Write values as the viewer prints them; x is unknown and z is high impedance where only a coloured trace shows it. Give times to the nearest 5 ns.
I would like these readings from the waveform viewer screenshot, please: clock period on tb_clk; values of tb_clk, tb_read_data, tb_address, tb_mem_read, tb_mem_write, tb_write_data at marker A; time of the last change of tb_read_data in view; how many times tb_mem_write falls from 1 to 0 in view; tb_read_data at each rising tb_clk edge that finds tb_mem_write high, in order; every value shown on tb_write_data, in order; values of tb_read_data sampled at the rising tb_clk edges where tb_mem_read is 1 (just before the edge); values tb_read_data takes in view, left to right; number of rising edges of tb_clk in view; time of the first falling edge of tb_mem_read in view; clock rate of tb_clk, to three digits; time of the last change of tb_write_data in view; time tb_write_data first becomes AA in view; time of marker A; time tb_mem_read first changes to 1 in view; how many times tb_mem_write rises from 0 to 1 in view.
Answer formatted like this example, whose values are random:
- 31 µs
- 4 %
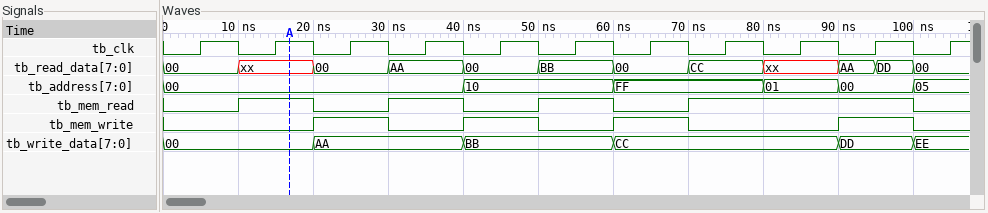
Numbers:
- 10 ns
- tb_clk=1, tb_read_data=xx, tb_address=00, tb_mem_read=1, tb_mem_write=0, tb_write_data=00
- 100 ns
- 4
- 00, 00, 00, AA
- 00, AA, BB, CC, DD, EE
- xx, AA, BB, CC, xx, AA
- 00, xx, 00, AA, 00, BB, 00, CC, xx, AA, DD, 00
- 11
- 20 ns
- 100 MHz
- 100 ns
- 20 ns
- 15 ns
- 10 ns
- 4
